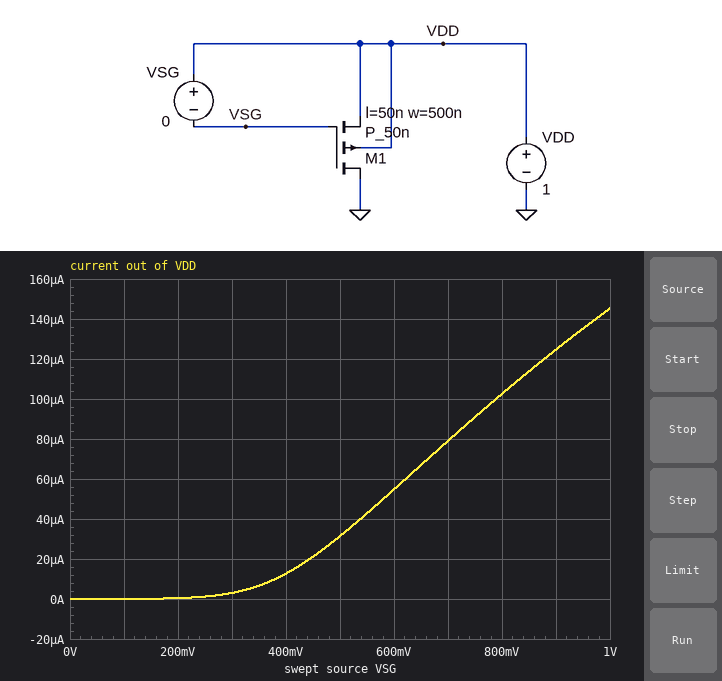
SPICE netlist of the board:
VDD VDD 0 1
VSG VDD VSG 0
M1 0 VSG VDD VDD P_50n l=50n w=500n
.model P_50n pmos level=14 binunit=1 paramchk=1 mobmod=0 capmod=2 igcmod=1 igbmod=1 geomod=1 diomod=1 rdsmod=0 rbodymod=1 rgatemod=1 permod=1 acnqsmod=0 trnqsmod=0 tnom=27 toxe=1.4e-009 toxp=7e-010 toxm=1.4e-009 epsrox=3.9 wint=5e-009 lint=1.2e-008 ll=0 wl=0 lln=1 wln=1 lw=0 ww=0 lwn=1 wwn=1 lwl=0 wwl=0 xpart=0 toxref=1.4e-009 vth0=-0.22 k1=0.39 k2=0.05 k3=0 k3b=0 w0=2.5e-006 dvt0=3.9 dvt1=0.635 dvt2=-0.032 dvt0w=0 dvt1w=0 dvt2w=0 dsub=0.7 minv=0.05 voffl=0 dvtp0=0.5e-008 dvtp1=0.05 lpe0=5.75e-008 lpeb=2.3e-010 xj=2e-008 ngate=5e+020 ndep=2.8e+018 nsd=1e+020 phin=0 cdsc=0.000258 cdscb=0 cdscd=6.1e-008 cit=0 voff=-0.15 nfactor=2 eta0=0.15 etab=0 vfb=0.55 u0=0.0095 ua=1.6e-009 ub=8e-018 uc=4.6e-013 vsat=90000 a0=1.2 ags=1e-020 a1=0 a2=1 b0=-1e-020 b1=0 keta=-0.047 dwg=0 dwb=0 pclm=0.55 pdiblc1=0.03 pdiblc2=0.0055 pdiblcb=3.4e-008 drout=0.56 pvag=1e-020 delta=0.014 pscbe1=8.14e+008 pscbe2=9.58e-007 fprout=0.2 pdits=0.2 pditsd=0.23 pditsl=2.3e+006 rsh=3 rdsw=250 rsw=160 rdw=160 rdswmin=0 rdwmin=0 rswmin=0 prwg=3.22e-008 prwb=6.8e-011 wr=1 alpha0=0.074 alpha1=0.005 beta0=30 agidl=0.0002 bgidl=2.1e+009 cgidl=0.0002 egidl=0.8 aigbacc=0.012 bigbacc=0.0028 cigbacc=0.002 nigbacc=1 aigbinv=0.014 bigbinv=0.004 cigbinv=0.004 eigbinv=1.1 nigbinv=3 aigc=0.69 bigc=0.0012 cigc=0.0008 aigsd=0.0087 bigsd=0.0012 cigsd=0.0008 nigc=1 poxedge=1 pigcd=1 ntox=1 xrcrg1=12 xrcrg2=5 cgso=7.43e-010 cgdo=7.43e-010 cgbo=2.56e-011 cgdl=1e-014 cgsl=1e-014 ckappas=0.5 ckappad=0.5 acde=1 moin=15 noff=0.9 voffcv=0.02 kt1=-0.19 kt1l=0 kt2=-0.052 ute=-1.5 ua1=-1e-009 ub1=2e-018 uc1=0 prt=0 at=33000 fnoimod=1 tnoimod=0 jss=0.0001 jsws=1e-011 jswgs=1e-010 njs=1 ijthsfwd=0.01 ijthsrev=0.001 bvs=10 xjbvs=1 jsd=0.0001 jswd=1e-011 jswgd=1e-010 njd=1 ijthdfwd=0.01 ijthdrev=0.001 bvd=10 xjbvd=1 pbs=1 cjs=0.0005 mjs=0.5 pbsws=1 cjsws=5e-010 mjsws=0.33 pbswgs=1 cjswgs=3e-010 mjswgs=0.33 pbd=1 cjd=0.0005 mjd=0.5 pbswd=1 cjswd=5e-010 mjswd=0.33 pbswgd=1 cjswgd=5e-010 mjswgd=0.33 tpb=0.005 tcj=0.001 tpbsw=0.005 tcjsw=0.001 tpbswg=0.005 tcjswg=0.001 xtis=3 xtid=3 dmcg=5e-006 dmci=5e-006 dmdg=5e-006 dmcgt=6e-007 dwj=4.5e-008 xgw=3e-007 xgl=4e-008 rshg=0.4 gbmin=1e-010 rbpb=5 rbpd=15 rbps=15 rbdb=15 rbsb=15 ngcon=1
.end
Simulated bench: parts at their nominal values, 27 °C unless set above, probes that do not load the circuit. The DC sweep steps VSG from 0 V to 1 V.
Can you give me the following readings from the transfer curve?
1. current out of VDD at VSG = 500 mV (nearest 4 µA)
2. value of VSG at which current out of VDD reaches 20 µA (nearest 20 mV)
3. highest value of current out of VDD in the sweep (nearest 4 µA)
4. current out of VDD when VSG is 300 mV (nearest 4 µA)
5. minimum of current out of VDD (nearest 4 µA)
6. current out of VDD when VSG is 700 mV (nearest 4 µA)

32 µA
440 mV
144 µA
4 µA
0 A
80 µA
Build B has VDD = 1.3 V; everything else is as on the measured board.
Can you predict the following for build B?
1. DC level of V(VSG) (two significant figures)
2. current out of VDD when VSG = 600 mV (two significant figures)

1.3 V
65 µA
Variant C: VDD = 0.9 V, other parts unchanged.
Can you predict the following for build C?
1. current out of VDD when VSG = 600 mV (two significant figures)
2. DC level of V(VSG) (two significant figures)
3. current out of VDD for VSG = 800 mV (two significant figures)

52 µA
900 mV
98 µA
